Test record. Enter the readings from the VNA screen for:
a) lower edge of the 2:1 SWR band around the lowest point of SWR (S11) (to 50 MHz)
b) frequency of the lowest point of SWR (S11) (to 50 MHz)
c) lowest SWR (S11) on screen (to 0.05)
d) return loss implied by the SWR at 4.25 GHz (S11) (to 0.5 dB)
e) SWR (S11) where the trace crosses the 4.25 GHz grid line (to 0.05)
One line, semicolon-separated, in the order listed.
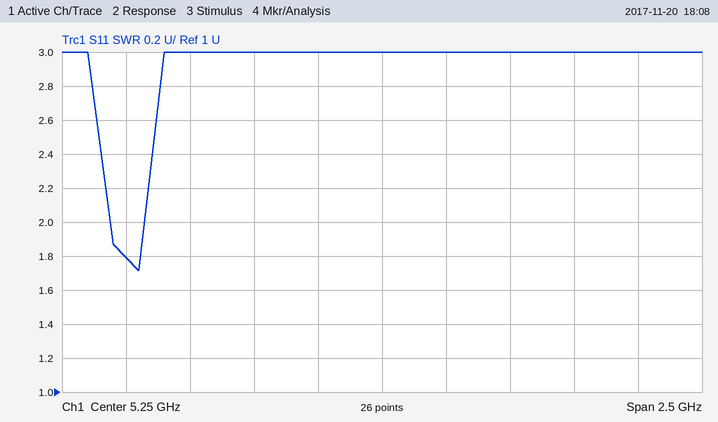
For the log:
4.20 GHz; 4.30 GHz; 1.70; 11.0 dB; 1.80
